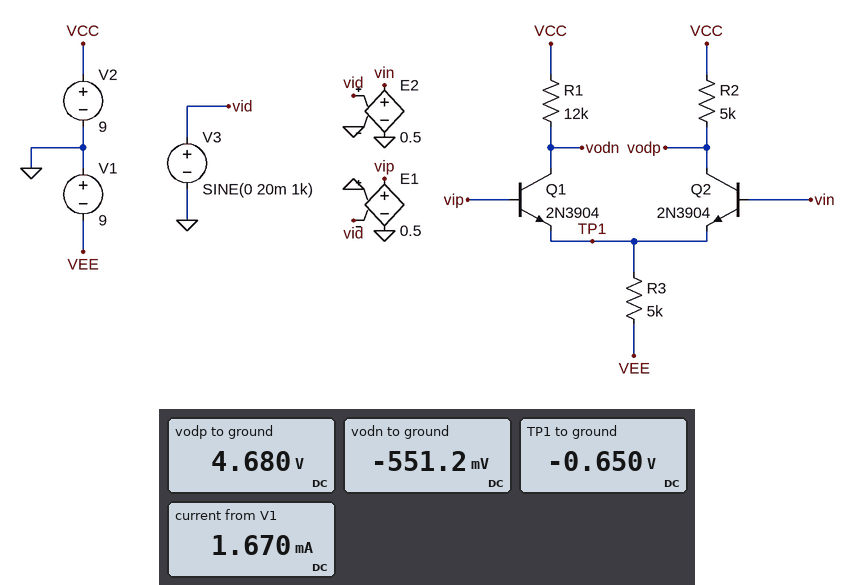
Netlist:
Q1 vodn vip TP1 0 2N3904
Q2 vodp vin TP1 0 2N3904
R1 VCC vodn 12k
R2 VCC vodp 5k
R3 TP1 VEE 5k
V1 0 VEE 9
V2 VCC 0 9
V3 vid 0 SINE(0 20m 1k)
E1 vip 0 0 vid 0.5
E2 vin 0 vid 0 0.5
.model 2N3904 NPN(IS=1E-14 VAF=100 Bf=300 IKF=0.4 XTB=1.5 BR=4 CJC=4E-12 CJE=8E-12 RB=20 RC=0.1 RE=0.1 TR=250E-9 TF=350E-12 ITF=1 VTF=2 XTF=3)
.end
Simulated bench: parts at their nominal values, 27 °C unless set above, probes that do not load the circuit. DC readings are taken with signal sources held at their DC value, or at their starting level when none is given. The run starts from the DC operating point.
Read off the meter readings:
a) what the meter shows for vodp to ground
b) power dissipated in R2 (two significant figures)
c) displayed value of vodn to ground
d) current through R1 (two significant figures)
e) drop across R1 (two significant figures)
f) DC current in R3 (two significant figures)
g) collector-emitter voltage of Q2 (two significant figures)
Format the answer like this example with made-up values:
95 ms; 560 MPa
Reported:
4.680 V; 3.7 mW; -551.2 mV; 800 µA; 9.6 V; 1.7 mA; 5.3 V
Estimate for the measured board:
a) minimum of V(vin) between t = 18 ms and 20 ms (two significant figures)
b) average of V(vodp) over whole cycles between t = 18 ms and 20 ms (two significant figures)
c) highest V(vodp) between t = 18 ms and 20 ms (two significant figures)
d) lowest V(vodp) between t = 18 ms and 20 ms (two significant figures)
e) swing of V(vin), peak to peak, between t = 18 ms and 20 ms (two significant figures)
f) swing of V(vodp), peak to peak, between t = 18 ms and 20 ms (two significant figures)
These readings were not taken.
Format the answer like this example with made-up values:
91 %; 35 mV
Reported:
-10 mV; 4.4 V; 5.3 V; 3.3 V; 20 mV; 2.0 V
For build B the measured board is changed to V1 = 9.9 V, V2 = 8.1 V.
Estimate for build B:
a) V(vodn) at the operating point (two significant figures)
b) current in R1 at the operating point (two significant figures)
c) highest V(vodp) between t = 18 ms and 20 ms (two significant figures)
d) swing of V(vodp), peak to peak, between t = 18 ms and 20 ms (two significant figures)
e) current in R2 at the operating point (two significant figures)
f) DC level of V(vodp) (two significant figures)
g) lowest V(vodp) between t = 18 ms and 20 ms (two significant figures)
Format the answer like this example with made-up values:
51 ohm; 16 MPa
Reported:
-620 mV; 730 µA; 3.5 V; 1.7 V; 1.1 mA; 2.8 V; 1.8 V
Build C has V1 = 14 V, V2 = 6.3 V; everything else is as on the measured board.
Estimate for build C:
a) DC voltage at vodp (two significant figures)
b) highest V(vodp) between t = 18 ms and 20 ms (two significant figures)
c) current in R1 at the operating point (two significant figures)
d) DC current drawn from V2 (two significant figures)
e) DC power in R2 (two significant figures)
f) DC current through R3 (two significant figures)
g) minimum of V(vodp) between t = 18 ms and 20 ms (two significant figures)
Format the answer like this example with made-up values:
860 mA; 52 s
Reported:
-660 mV; -650 mV; 580 µA; 2.0 mA; 9.7 mW; 2.7 mA; -670 mV
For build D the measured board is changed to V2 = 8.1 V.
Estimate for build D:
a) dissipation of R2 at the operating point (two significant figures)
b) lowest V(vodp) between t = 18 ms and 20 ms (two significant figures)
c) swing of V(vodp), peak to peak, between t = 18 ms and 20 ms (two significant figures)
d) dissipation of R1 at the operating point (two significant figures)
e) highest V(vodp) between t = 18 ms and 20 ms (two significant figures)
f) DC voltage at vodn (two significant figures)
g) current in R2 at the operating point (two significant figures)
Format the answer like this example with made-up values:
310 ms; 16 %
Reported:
4.2 mW; 2.4 V; 1.8 V; 6.3 mW; 4.2 V; -600 mV; 910 µA
